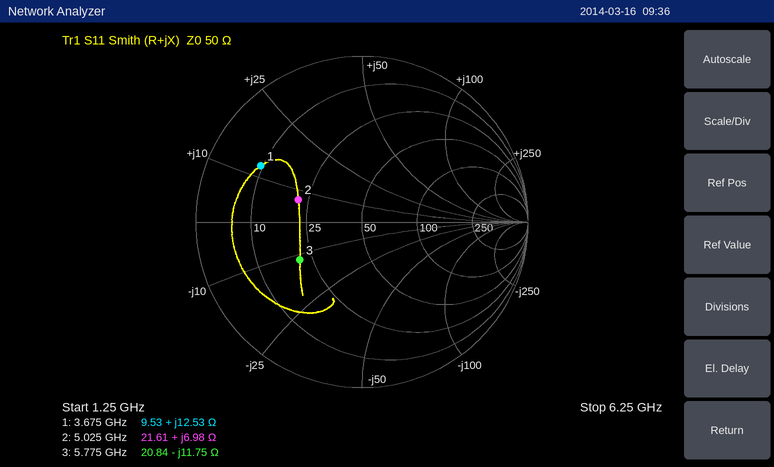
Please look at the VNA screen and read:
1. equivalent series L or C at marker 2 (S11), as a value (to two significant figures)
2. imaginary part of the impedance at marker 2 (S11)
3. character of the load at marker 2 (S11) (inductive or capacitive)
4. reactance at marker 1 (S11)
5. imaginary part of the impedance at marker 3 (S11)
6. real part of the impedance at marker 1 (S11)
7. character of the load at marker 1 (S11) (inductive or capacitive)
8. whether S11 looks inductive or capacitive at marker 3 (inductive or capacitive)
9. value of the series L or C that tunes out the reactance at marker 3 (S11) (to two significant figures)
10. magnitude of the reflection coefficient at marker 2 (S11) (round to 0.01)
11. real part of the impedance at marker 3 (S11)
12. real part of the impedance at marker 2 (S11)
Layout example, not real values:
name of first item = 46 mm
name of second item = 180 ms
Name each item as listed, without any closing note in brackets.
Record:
equivalent series L or C at marker 2 (S11), as a value = 220 pH
imaginary part of the impedance at marker 2 = +6.98 Ω
character of the load at marker 2 (S11) = inductive
reactance at marker 1 = +12.53 Ω
imaginary part of the impedance at marker 3 = -11.75 Ω
real part of the impedance at marker 1 = 9.53 Ω
character of the load at marker 1 (S11) = inductive
whether S11 looks inductive or capacitive at marker 3 = capacitive
value of the series L or C that tunes out the reactance at marker 3 (S11) = 320 pH
magnitude of the reflection coefficient at marker 2 (S11) = 0.41
real part of the impedance at marker 3 = 20.84 Ω
real part of the impedance at marker 2 = 21.61 Ω
